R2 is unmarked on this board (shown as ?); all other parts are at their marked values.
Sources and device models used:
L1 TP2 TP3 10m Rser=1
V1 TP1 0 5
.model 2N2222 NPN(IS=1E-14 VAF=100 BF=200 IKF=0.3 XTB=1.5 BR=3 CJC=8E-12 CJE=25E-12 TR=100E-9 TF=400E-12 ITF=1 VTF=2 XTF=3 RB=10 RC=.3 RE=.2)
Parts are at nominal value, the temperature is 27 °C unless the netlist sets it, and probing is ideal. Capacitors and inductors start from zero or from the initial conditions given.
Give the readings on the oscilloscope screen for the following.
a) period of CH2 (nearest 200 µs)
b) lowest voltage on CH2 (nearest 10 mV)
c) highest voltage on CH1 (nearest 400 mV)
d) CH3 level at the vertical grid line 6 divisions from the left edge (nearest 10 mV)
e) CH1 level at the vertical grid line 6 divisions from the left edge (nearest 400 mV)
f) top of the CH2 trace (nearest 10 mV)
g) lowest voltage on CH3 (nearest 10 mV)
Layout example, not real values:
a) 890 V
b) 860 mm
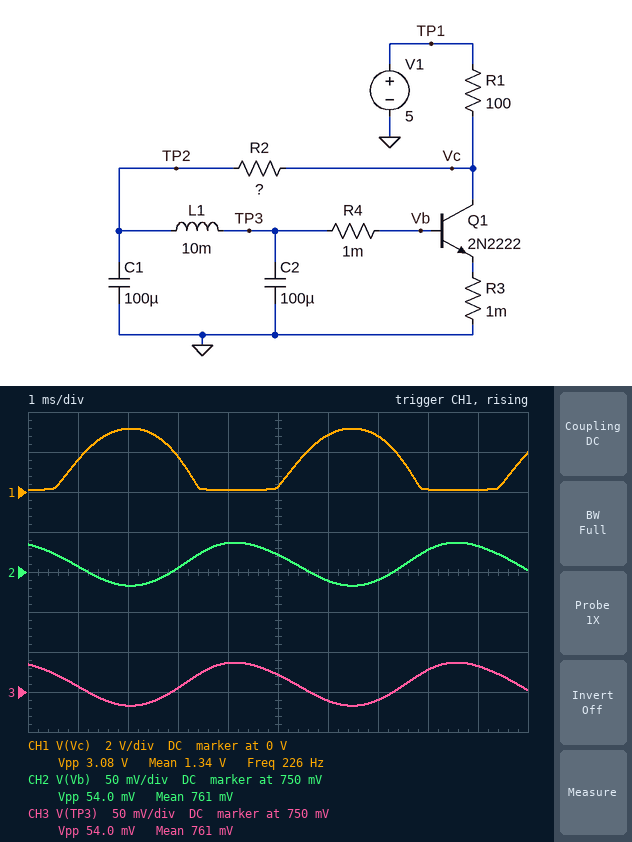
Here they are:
a) 4.4 ms
b) 730 mV
c) 3.2 V
d) 740 mV
e) 2.8 V
f) 790 mV
g) 730 mV
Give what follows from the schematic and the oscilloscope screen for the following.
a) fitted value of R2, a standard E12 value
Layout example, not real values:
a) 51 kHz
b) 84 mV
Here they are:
a) 1.5 kΩ
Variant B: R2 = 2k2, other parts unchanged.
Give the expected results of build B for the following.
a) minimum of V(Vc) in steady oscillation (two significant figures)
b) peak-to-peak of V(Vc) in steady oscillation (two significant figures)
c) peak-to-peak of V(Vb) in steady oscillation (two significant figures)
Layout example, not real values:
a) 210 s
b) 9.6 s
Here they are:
a) 120 mV
b) 2.7 V
c) 39 mV
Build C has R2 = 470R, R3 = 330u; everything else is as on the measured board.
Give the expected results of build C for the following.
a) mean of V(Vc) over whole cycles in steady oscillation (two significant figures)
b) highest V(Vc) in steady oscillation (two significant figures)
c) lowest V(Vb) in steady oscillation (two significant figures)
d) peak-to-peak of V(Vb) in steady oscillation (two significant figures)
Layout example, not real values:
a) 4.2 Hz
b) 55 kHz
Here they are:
a) 1.7 V
b) 4.0 V
c) 680 mV
d) 160 mV
